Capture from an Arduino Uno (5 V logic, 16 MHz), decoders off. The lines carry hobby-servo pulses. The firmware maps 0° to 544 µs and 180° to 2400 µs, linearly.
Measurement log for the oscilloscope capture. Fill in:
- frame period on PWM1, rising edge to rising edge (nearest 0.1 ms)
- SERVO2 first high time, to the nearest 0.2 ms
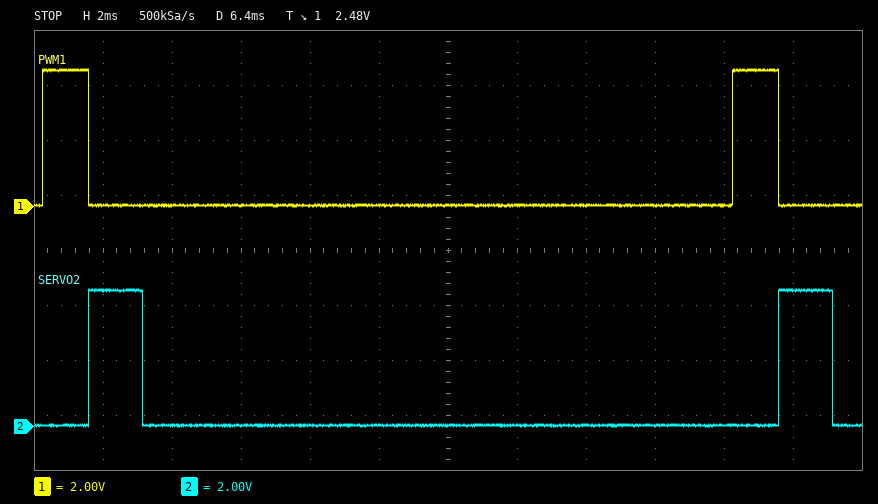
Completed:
20.0 ms
1.6 ms
